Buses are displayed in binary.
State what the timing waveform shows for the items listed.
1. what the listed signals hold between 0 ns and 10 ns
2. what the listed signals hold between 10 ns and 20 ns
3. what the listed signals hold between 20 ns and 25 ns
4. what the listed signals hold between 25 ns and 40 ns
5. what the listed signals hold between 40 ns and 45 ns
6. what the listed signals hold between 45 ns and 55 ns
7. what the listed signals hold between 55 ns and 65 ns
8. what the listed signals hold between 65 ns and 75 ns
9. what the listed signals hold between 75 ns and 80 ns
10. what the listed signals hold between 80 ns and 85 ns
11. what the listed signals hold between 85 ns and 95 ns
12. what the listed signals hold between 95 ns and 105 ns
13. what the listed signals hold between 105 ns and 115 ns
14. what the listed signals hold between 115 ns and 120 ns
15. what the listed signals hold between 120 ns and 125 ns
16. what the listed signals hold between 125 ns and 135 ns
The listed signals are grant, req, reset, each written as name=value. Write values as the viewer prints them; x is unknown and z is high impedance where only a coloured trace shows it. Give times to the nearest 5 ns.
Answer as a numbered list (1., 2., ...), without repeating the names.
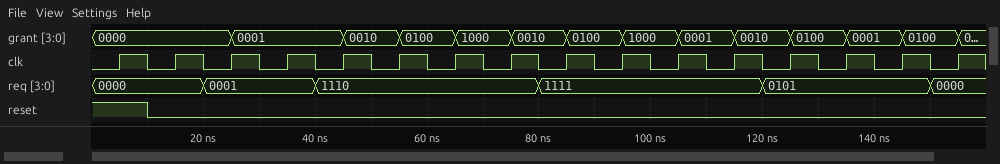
1. grant=0000, req=0000, reset=1
2. grant=0000, req=0000, reset=0
3. grant=0000, req=0001, reset=0
4. grant=0001, req=0001, reset=0
5. grant=0001, req=1110, reset=0
6. grant=0010, req=1110, reset=0
7. grant=0100, req=1110, reset=0
8. grant=1000, req=1110, reset=0
9. grant=0010, req=1110, reset=0
10. grant=0010, req=1111, reset=0
11. grant=0100, req=1111, reset=0
12. grant=1000, req=1111, reset=0
13. grant=0001, req=1111, reset=0
14. grant=0010, req=1111, reset=0
15. grant=0010, req=0101, reset=0
16. grant=0100, req=0101, reset=0
